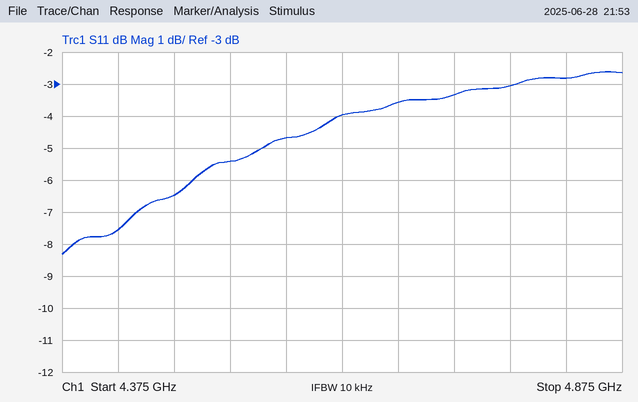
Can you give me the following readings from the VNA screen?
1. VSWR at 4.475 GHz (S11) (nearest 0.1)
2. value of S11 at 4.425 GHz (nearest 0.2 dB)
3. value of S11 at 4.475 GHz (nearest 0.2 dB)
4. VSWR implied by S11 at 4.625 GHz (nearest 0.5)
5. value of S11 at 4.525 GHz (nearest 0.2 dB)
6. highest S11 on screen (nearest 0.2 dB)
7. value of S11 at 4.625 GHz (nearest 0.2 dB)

2.8
-7.6 dB
-6.4 dB
4.5
-5.4 dB
-2.6 dB
-4.0 dB
